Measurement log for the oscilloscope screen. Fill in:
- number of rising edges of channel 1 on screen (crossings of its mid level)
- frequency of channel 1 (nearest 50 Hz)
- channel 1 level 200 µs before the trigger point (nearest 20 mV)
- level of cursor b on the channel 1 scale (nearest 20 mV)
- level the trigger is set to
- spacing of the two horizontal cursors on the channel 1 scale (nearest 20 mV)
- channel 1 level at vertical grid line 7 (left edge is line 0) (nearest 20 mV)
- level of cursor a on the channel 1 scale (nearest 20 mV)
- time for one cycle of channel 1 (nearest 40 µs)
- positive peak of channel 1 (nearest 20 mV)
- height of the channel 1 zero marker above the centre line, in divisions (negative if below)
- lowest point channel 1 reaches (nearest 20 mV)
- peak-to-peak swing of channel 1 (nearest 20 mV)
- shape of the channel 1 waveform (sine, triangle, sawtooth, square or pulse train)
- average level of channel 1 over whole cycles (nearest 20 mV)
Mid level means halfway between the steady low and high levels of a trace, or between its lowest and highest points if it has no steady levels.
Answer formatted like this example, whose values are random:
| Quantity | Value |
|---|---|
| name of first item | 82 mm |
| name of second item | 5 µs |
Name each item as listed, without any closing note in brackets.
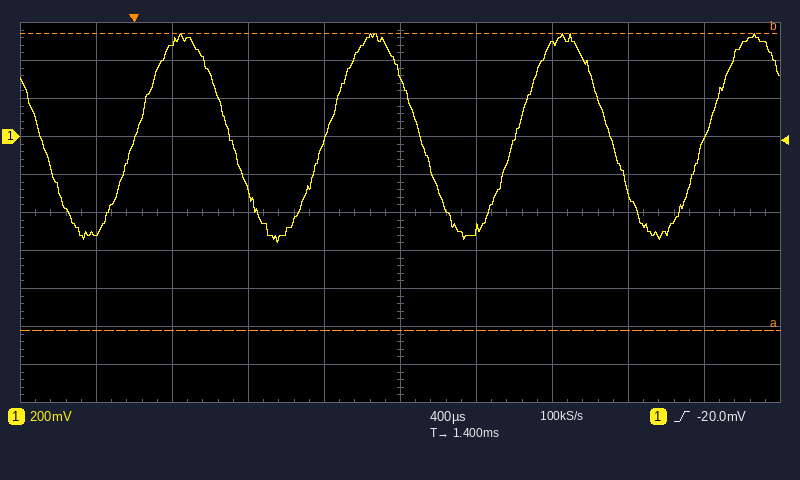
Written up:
| Quantity | Value |
|---|---|
| number of rising edges of channel 1 on screen | 4 |
| frequency of channel 1 | 1.00 kHz |
| channel 1 level 200 µs before the trigger point | -500 mV |
| level of cursor b on the channel 1 scale | 540 mV |
| level the trigger is set to | -20.0 mV |
| spacing of the two horizontal cursors on the channel 1 scale | 1.56 V |
| channel 1 level at vertical grid line 7 (left edge is line 0) | 480 mV |
| level of cursor a on the channel 1 scale | -1.02 V |
| time for one cycle of channel 1 | 1.00 ms |
| positive peak of channel 1 | 540 mV |
| height of the channel 1 zero marker above the centre line, in divisions | +2.0 div |
| lowest point channel 1 reaches | -560 mV |
| peak-to-peak swing of channel 1 | 1.10 V |
| shape of the channel 1 waveform | sine |
| average level of channel 1 over whole cycles | 0 mV |
